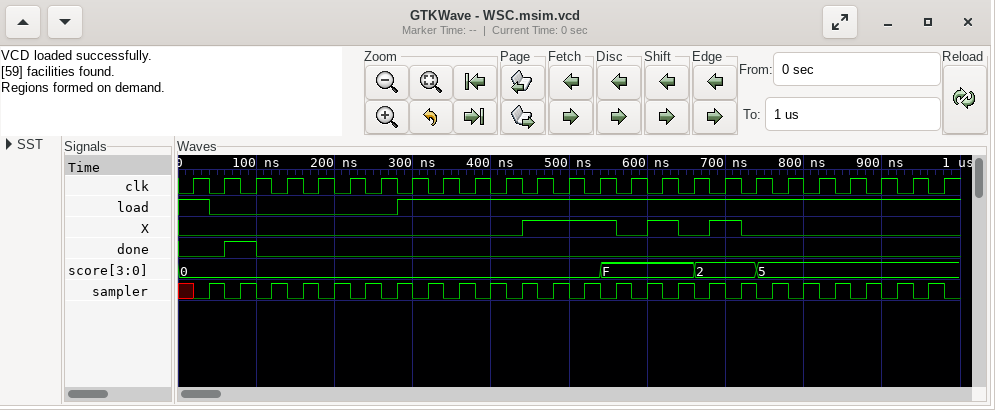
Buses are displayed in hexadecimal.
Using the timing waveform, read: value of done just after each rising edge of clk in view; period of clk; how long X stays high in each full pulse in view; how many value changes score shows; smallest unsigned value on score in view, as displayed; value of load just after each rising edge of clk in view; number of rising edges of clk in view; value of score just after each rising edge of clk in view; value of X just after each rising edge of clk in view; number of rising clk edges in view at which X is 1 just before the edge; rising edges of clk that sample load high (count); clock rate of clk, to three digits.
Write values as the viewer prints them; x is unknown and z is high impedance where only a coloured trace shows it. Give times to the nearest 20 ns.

0 1 0 0 0 0 0 0 0 0 0 0 0 0 0 0 0 0 0 0 0 0 0 0 0
40 ns
120 ns, 40 ns, 40 ns
3
0
1 0 0 0 0 0 0 1 1 1 1 1 1 1 1 1 1 1 1 1 1 1 1 1 1
25
0, 0, 0, 0, 0, 0, 0, 0, 0, 0, 0, 0, 0, F, F, F, 2, 2, 5, 5, 5, 5, 5, 5, 5
0 0 0 0 0 0 0 0 0 0 0 1 1 1 0 1 0 1 0 0 0 0 0 0 0
5
19
25.0 MHz
